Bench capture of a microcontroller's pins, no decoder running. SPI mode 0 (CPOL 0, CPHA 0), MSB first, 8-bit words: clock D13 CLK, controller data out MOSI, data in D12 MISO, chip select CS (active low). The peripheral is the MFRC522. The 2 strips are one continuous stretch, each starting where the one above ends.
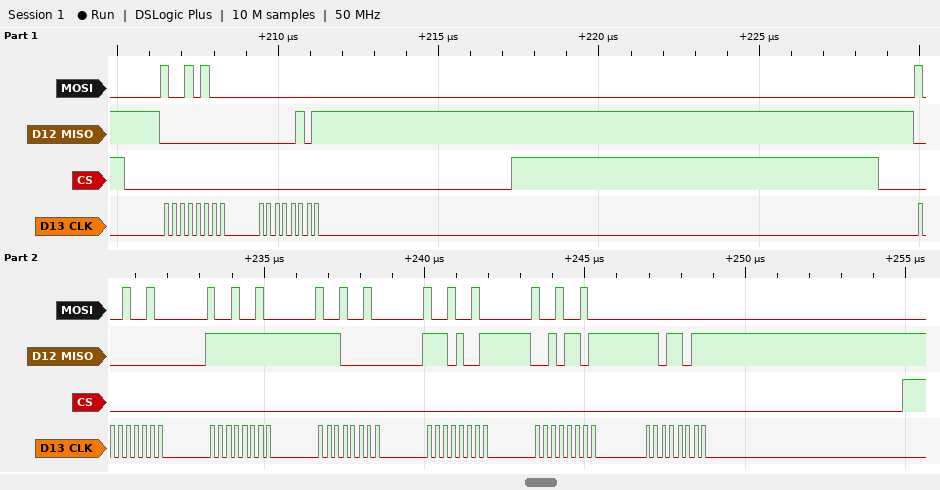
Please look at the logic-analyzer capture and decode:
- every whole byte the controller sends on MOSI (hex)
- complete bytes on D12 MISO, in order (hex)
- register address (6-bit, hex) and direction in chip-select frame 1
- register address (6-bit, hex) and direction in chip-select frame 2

0x94 0x00 0x92 0x92 0x92 0x92 0x92 0x00
0x00 0x05 0x00 0xFF 0xE0 0xE9 0x2D 0xDB
0x0A read
0x09 read
